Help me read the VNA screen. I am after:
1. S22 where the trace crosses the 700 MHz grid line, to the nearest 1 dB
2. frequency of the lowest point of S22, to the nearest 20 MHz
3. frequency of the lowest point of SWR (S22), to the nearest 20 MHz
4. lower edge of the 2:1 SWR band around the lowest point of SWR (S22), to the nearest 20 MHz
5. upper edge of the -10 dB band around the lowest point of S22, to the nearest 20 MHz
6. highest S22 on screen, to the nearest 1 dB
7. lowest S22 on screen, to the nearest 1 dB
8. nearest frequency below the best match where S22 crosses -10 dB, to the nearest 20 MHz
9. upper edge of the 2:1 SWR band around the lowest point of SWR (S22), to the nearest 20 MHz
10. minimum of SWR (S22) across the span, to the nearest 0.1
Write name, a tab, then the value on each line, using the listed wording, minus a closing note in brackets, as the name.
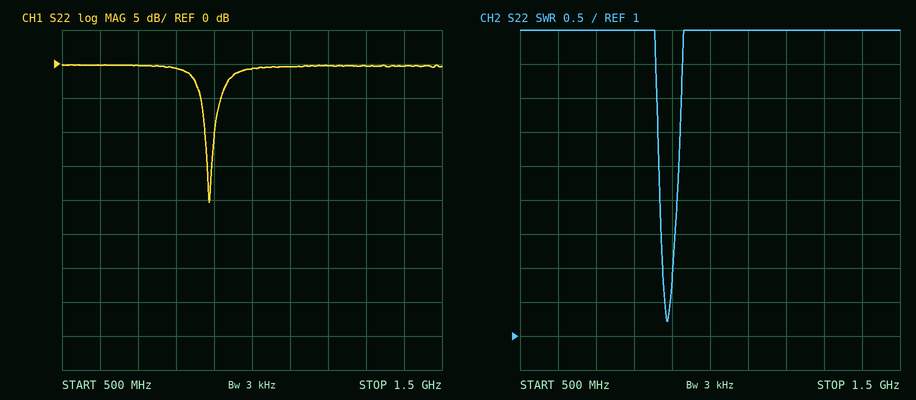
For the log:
S22 where the trace crosses the 700 MHz grid line, to the nearest 1 dB	0 dB
frequency of the lowest point of S22, to the nearest 20 MHz	880 MHz
frequency of the lowest point of SWR (S22), to the nearest 20 MHz	880 MHz
lower edge of the 2:1 SWR band around the lowest point of SWR (S22), to the nearest 20 MHz	880 MHz
upper edge of the -10 dB band around the lowest point of S22, to the nearest 20 MHz	900 MHz
highest S22 on screen, to the nearest 1 dB	0 dB
lowest S22 on screen, to the nearest 1 dB	-20 dB
nearest frequency below the best match where S22 crosses -10 dB, to the nearest 20 MHz	880 MHz
upper edge of the 2:1 SWR band around the lowest point of SWR (S22), to the nearest 20 MHz	900 MHz
minimum of SWR (S22) across the span, to the nearest 0.1	1.2
